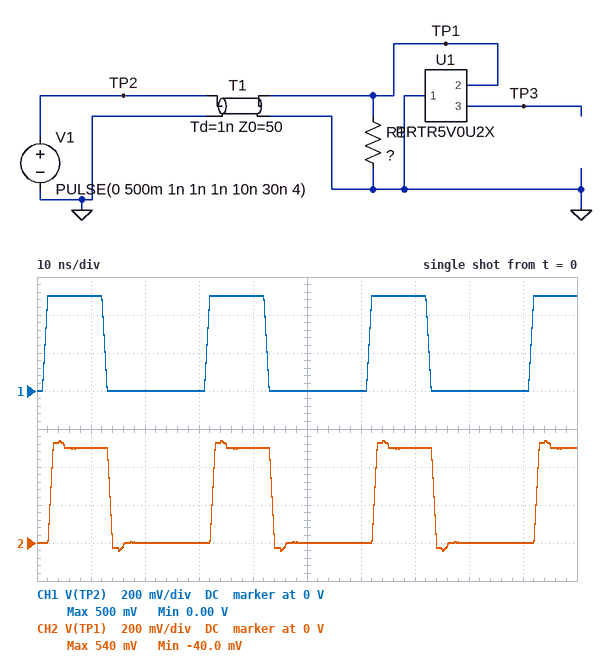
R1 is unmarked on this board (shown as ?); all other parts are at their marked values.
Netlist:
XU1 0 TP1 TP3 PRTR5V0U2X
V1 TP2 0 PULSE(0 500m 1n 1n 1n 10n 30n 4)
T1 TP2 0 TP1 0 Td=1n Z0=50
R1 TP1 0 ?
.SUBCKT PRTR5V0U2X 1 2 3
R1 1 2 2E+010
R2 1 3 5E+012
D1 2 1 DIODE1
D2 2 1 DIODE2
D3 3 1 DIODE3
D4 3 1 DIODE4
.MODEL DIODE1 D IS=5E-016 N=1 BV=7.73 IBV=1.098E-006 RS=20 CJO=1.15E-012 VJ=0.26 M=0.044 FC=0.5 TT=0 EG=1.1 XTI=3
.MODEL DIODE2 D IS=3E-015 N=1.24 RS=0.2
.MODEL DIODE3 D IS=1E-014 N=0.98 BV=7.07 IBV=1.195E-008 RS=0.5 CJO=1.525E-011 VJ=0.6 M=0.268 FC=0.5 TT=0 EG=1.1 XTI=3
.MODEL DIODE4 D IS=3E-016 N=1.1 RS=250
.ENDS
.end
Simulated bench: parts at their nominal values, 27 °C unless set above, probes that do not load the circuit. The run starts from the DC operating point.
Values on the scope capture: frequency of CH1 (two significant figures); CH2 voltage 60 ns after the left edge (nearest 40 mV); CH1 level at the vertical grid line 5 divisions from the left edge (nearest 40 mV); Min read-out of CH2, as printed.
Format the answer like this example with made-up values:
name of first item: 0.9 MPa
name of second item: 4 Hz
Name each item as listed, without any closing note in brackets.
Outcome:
frequency of CH1: 33 MHz
CH2 voltage 60 ns after the left edge: 0 V
CH1 level at the vertical grid line 5 divisions from the left edge: 0 V
Min read-out of CH2, as printed: -40.0 mV
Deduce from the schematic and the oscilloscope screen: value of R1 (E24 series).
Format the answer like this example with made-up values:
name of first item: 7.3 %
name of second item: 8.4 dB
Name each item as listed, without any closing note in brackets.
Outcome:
value of R1: 56 Ω
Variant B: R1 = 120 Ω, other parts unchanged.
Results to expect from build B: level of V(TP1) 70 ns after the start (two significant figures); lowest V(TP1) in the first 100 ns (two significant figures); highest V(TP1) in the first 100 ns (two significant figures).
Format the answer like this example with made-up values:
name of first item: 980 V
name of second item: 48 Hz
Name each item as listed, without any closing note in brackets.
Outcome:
level of V(TP1) 70 ns after the start: 490 mV
lowest V(TP1) in the first 100 ns: -210 mV
highest V(TP1) in the first 100 ns: 700 mV
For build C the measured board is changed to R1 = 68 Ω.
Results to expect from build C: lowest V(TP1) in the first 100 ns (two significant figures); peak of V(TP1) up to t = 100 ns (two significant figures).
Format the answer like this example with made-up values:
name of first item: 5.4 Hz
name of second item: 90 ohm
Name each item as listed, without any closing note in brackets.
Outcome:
lowest V(TP1) in the first 100 ns: -86 mV
peak of V(TP1) up to t = 100 ns: 580 mV
